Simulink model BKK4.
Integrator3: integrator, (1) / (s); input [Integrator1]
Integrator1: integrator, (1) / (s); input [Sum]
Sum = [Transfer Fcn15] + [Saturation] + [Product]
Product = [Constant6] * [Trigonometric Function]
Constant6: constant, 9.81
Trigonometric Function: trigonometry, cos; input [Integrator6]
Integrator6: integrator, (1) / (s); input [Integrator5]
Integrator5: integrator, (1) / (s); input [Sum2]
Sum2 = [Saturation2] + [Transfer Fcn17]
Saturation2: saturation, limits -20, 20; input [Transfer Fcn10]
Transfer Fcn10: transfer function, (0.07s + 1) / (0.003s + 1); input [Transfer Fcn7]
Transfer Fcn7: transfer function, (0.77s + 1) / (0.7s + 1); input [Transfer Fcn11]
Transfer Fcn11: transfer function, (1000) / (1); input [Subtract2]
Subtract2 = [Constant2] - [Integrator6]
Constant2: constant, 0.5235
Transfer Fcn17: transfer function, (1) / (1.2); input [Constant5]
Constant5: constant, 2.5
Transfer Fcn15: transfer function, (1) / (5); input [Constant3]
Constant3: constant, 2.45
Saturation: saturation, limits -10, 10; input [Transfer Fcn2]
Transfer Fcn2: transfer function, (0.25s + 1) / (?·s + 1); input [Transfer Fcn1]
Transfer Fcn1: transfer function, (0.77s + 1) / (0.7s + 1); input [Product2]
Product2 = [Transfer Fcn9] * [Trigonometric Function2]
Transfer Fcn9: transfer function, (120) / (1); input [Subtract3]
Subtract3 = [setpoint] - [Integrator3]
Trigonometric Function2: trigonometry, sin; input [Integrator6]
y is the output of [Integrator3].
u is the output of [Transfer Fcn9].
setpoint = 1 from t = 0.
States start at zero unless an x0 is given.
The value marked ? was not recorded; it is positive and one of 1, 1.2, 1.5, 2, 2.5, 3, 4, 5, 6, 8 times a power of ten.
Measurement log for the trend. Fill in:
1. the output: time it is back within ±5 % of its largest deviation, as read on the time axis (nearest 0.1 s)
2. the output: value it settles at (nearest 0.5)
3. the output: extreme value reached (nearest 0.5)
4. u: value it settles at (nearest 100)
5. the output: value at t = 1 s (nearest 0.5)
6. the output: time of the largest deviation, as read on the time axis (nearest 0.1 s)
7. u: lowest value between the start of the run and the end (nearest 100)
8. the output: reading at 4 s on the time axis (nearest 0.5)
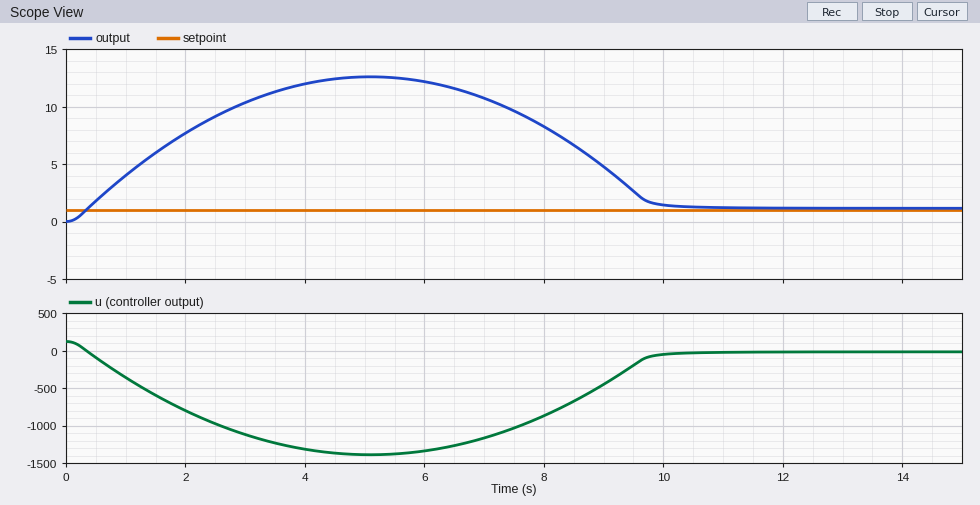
9.7 s
1.0
12.5
0
4.0
5.1 s
-1400
12.0
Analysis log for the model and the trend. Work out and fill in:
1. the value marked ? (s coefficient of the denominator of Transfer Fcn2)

0.04
